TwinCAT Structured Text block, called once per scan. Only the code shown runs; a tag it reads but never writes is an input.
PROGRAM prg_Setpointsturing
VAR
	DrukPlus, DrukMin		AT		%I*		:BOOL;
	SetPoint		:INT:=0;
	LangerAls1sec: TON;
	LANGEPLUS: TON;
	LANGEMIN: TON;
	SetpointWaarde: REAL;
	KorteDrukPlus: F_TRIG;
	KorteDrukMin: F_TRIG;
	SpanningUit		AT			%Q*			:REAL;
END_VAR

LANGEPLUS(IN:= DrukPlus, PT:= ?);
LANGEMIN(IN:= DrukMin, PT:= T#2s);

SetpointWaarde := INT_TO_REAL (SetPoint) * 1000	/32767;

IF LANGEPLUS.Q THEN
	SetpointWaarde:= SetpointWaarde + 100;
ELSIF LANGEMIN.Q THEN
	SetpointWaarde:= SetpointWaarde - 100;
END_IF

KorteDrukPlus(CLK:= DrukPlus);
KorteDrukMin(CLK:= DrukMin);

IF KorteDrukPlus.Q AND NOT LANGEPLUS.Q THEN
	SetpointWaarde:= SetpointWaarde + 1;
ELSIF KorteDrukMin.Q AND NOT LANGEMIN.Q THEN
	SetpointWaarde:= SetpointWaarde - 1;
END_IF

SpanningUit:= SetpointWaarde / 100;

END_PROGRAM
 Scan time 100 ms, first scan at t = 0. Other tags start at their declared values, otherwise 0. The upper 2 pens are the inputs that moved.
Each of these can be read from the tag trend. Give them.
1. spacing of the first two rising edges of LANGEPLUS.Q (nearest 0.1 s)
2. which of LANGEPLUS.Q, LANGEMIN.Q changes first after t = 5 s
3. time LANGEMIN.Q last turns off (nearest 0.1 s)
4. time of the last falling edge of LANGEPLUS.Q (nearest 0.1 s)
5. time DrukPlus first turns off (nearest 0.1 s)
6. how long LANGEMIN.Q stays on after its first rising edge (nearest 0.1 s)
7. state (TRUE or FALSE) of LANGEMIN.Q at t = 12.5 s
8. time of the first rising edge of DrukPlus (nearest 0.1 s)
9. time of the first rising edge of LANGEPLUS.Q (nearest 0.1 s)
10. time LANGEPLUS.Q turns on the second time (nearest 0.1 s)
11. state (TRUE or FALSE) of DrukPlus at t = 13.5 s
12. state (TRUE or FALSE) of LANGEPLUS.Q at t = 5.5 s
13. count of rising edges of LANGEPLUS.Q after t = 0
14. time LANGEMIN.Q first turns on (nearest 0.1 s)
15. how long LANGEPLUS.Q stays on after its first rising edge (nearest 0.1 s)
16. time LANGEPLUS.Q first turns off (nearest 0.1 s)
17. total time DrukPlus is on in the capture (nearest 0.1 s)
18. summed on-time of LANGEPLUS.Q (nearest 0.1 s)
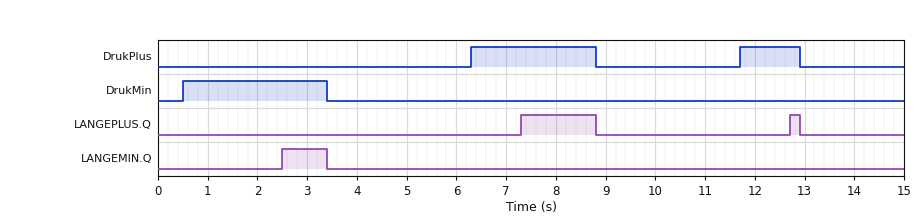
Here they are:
5.4 s
LANGEPLUS.Q
3.4 s
12.9 s
8.8 s
0.9 s
FALSE
6.3 s
7.3 s
12.7 s
FALSE
FALSE
2
2.5 s
1.5 s
8.8 s
3.7 s
1.7 s
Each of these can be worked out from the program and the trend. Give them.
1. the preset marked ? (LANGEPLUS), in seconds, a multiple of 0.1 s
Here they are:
1.0 s
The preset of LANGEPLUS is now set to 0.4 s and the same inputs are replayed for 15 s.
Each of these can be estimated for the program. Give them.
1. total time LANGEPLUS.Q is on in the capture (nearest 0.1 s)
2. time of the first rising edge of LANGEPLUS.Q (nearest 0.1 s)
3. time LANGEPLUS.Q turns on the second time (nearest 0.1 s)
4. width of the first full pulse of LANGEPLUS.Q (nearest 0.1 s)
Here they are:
2.9 s
6.7 s
12.1 s
2.1 s
